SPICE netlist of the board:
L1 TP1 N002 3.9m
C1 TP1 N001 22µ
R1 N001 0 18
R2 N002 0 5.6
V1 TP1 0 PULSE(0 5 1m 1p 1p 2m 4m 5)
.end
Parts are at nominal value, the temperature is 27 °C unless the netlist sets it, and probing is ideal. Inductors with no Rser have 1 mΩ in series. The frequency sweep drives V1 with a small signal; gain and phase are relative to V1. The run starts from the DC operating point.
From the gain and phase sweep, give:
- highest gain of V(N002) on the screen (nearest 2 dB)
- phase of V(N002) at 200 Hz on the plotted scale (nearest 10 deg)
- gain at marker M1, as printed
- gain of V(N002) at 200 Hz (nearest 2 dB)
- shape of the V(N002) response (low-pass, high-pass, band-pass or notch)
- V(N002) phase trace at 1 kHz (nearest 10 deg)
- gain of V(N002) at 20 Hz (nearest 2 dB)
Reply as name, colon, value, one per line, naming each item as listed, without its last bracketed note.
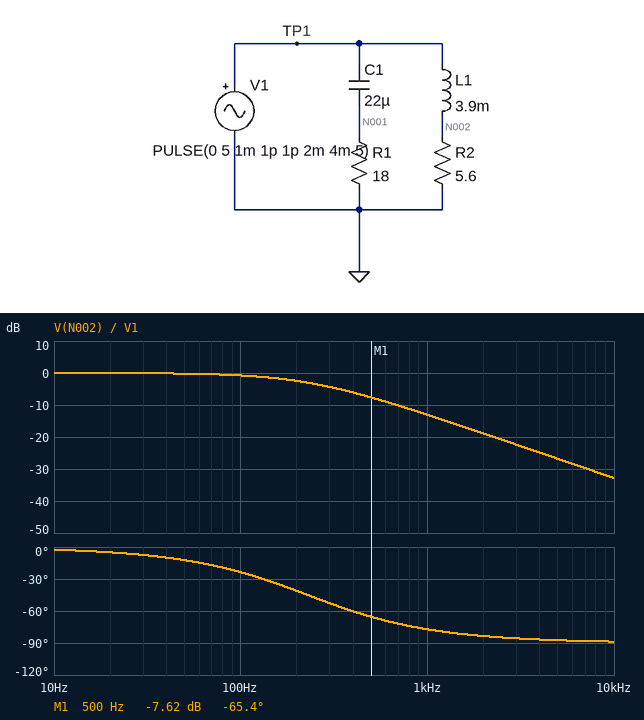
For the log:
highest gain of V(N002) on the screen: 0 dB
phase of V(N002) at 200 Hz on the plotted scale: -40 deg
gain at marker M1, as printed: -7.62 dB
gain of V(N002) at 200 Hz: -2 dB
shape of the V(N002) response: low-pass
V(N002) phase trace at 1 kHz: -80 deg
gain of V(N002) at 20 Hz: 0 dB
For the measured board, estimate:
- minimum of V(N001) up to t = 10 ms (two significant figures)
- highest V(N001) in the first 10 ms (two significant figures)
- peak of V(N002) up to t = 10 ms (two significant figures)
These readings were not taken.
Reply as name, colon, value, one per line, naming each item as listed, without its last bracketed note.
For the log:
minimum of V(N001) up to t = 10 ms: -5.0 V
highest V(N001) in the first 10 ms: 5.0 V
peak of V(N002) up to t = 10 ms: 4.7 V
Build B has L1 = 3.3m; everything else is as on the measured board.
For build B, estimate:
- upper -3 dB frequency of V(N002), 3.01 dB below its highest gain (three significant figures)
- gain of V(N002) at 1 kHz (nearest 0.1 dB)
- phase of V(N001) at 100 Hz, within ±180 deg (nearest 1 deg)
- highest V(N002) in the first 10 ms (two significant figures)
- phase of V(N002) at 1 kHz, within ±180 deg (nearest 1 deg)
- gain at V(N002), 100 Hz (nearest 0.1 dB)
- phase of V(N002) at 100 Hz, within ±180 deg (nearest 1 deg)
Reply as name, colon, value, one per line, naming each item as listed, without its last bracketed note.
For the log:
upper -3 dB frequency of V(N002), 3.01 dB below its highest gain: 270 Hz
gain of V(N002) at 1 kHz: -11.7 dB
phase of V(N001) at 100 Hz, within ±180 deg: 76 deg
highest V(N002) in the first 10 ms: 4.8 V
phase of V(N002) at 1 kHz, within ±180 deg: -75 deg
gain at V(N002), 100 Hz: -0.6 dB
phase of V(N002) at 100 Hz, within ±180 deg: -20 deg
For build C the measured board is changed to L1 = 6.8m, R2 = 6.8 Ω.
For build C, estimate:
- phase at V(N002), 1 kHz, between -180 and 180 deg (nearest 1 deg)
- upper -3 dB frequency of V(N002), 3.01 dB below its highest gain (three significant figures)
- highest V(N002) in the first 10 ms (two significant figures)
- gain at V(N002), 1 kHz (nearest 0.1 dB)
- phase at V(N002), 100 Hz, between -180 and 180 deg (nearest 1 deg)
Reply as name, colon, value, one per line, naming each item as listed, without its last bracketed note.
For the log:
phase at V(N002), 1 kHz, between -180 and 180 deg: -81 deg
upper -3 dB frequency of V(N002), 3.01 dB below its highest gain: 159 Hz
highest V(N002) in the first 10 ms: 4.4 V
gain at V(N002), 1 kHz: -16.1 dB
phase at V(N002), 100 Hz, between -180 and 180 deg: -32 deg
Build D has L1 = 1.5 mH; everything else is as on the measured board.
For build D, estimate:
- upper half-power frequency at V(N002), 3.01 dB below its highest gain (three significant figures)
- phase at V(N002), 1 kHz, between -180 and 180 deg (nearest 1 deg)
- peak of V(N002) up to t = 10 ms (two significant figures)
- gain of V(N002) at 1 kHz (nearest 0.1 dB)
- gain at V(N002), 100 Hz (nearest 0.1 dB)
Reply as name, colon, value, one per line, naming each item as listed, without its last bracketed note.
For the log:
upper half-power frequency at V(N002), 3.01 dB below its highest gain: 594 Hz
phase at V(N002), 1 kHz, between -180 and 180 deg: -59 deg
peak of V(N002) up to t = 10 ms: 5.0 V
gain of V(N002) at 1 kHz: -5.8 dB
gain at V(N002), 100 Hz: -0.1 dB
